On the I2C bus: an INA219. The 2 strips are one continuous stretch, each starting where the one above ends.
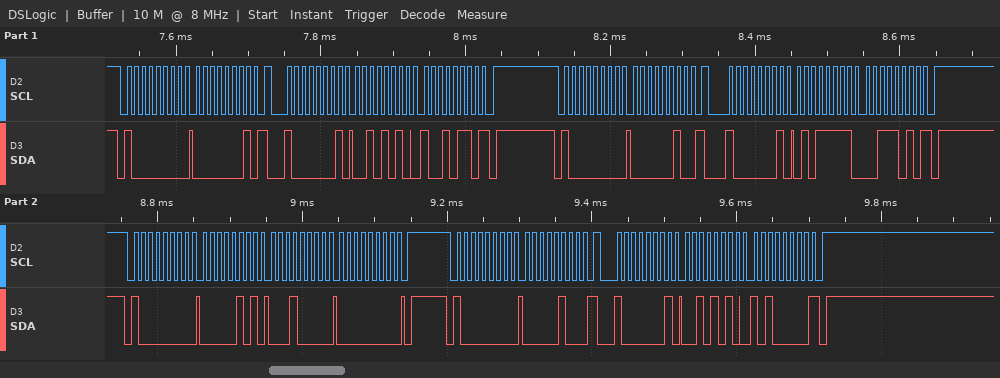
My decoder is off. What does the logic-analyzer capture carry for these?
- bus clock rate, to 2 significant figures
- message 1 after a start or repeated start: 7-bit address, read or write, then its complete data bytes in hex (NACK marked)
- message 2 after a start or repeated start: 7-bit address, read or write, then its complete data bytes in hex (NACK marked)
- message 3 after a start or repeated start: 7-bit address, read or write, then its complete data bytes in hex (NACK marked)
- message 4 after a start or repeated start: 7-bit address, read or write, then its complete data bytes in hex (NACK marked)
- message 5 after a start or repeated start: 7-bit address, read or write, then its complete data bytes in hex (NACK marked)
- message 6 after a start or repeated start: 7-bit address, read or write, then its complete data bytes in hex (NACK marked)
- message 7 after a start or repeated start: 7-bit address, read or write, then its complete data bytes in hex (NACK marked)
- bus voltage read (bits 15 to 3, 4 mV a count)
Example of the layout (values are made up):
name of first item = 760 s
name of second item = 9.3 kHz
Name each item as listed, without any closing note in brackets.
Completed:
bus clock rate, to 2 significant figures = 100 kHz
message 1 after a start or repeated start: 7-bit address, read or write, then its complete data bytes in hex = 0x40 write: 01
message 2 after a start or repeated start: 7-bit address, read or write, then its complete data bytes in hex = 0x40 read: 2A 96 NACK
message 3 after a start or repeated start: 7-bit address, read or write, then its complete data bytes in hex = 0x40 write: 02
message 4 after a start or repeated start: 7-bit address, read or write, then its complete data bytes in hex = 0x40 read: 5F 3A NACK
message 5 after a start or repeated start: 7-bit address, read or write, then its complete data bytes in hex = 0x40 write: 05 10 00
message 6 after a start or repeated start: 7-bit address, read or write, then its complete data bytes in hex = 0x40 write: 04
message 7 after a start or repeated start: 7-bit address, read or write, then its complete data bytes in hex = 0x40 read: 2A A0 NACK
bus voltage read = 12.188 V
